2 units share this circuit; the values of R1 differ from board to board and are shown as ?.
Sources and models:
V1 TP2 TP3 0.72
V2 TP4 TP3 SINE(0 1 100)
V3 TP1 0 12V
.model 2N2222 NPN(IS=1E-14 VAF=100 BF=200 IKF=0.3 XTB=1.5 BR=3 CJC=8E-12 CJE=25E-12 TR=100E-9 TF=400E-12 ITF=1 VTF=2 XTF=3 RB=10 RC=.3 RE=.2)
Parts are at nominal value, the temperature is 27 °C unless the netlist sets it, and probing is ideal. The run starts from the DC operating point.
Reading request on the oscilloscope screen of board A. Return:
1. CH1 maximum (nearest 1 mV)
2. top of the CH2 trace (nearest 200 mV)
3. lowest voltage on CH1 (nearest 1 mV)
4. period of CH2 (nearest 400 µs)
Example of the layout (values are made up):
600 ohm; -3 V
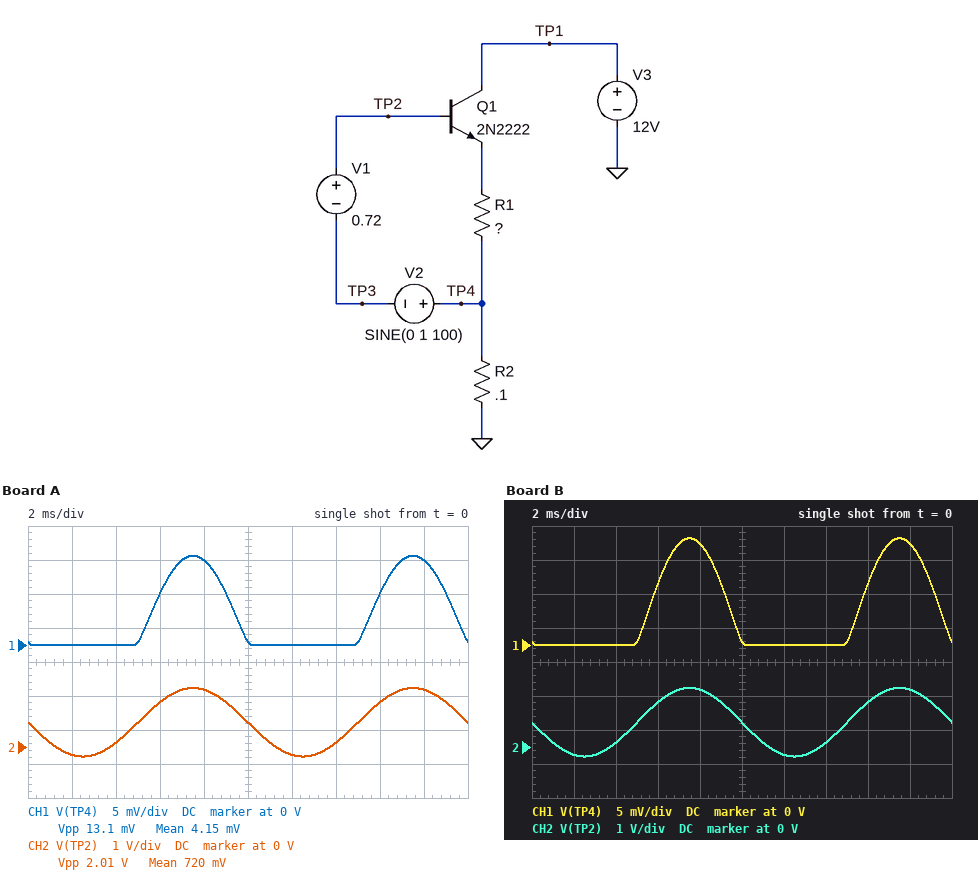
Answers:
13 mV; 1.8 V; 0 V; 10.0 ms
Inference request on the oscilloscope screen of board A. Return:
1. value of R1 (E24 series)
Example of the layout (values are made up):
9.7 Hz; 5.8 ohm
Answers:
6.8 Ω
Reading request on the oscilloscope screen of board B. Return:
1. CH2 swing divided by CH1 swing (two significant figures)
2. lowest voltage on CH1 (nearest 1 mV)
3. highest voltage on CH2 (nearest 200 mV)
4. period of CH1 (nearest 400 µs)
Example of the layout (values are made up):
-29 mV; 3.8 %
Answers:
130; 0 V; 1.8 V; 10.0 ms
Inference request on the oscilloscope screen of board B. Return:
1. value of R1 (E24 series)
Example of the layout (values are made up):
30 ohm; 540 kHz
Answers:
5.6 Ω
